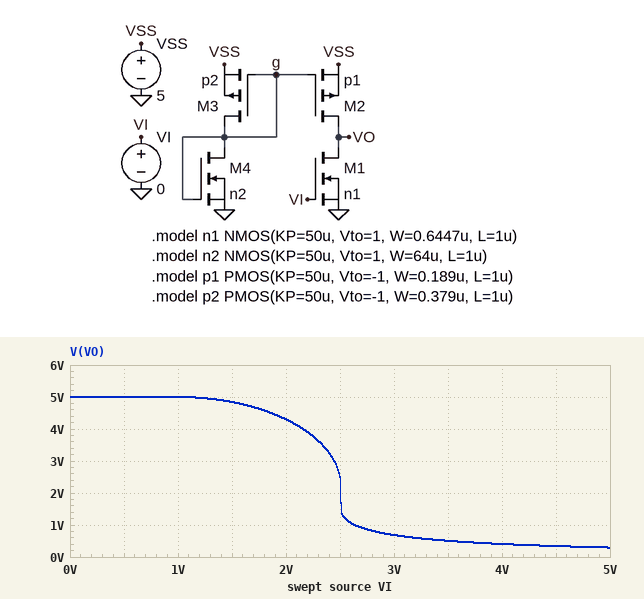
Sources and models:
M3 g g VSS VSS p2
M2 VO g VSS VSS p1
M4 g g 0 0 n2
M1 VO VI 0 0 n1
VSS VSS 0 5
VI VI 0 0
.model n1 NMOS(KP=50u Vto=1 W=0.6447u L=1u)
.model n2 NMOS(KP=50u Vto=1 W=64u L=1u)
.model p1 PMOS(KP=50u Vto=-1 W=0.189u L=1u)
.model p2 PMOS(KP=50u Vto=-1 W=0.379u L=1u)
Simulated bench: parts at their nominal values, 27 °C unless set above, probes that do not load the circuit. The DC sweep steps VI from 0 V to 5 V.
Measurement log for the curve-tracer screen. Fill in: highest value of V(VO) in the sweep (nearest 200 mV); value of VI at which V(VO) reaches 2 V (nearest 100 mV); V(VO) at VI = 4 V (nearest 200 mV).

5.0 V
2.5 V
400 mV
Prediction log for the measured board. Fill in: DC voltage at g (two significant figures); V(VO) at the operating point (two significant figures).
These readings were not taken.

1.2 V
5.0 V
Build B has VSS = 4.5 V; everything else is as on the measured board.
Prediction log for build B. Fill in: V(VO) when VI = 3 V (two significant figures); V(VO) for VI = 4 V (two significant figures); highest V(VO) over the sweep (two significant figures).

440 mV
280 mV
4.5 V
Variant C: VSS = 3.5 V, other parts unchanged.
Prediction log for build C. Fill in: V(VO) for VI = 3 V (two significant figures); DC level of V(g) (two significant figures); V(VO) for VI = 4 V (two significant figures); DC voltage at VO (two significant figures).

150 mV
1.1 V
96 mV
3.5 V
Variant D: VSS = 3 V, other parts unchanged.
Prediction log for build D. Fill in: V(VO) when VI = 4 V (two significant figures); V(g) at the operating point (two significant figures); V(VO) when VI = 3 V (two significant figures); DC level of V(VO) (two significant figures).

42 mV
1.1 V
64 mV
3.0 V
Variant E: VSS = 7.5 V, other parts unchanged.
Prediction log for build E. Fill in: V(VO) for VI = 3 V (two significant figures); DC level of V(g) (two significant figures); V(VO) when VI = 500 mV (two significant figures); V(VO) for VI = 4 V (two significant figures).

5.9 V
1.4 V
7.5 V
1.8 V
